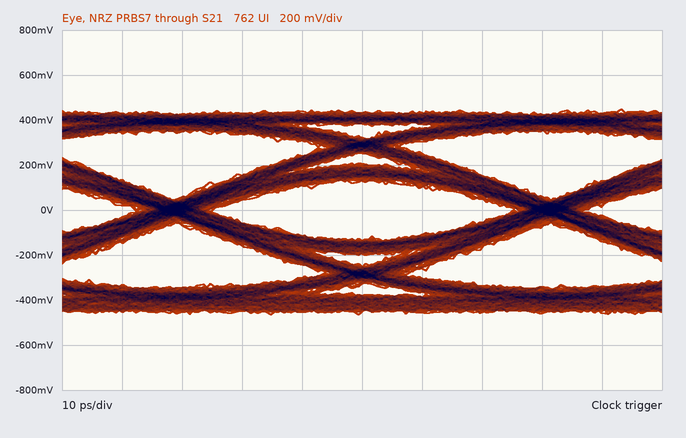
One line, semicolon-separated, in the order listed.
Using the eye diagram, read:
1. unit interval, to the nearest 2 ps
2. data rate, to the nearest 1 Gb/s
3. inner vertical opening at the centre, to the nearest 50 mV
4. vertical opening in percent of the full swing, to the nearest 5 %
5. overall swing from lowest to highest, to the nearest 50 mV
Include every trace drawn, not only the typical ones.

62 ps; 16 Gb/s; 250 mV; 30 %; 900 mV
